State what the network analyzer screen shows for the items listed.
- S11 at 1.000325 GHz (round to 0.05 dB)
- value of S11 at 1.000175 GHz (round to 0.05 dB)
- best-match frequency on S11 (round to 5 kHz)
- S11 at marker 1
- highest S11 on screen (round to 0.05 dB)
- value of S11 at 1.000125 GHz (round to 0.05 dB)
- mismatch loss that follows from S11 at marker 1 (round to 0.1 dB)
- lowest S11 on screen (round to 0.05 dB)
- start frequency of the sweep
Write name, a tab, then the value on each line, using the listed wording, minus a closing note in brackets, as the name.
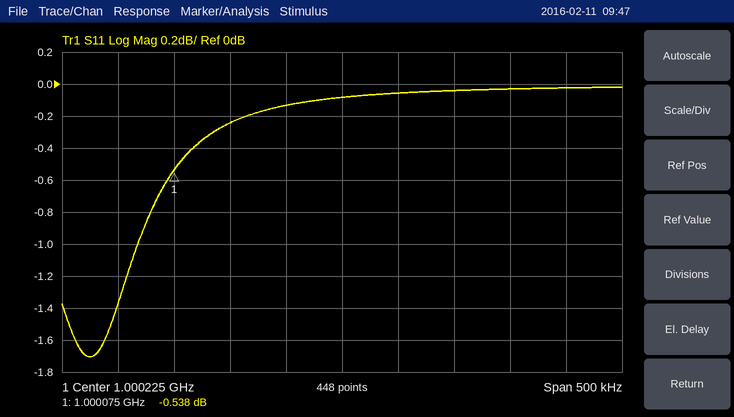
S11 at 1.000325 GHz	-0.05 dB
value of S11 at 1.000175 GHz	-0.15 dB
best-match frequency on S11	1.000000 GHz
S11 at marker 1	-0.538 dB
highest S11 on screen	0.00 dB
value of S11 at 1.000125 GHz	-0.25 dB
mismatch loss that follows from S11 at marker 1	9.3 dB
lowest S11 on screen	-1.70 dB
start frequency of the sweep	999.975 MHz
